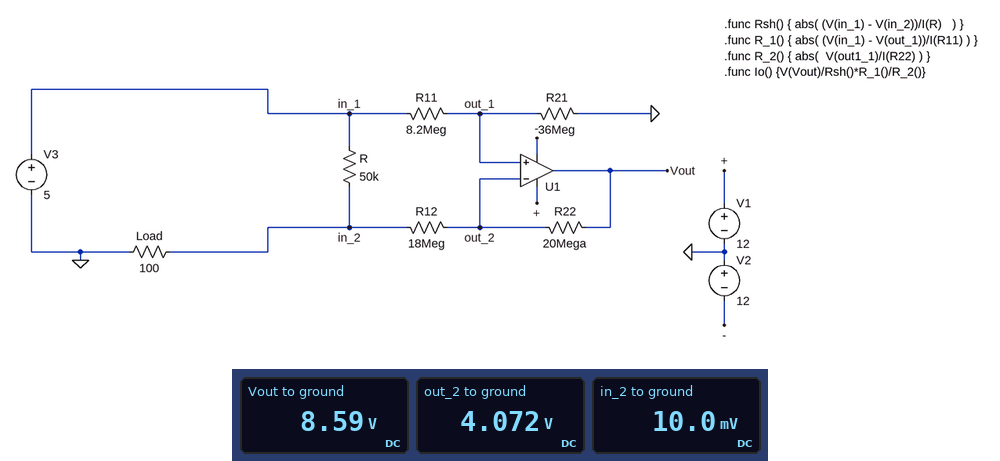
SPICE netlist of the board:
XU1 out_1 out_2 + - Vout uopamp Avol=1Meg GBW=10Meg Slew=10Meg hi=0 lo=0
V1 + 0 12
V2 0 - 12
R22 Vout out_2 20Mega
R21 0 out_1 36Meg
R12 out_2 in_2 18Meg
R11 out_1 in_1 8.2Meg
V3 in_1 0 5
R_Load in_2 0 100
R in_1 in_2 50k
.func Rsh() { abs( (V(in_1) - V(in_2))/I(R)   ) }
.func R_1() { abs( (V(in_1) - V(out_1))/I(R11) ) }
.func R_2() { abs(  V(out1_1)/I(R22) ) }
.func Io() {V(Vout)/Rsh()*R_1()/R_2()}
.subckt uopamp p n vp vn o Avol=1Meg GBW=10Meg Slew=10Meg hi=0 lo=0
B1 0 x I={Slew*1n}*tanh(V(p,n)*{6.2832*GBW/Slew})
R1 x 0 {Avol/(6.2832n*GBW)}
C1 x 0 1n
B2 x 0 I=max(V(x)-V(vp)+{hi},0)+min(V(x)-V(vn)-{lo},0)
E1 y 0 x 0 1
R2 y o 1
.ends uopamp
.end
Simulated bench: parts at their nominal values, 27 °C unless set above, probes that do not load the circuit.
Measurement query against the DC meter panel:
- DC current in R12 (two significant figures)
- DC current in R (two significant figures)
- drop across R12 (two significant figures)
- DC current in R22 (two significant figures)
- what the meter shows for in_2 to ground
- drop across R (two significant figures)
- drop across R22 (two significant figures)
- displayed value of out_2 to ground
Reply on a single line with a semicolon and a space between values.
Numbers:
230 nA; 100 µA; 4.1 V; 230 nA; 10.0 mV; 5.0 V; 4.5 V; 4.072 V
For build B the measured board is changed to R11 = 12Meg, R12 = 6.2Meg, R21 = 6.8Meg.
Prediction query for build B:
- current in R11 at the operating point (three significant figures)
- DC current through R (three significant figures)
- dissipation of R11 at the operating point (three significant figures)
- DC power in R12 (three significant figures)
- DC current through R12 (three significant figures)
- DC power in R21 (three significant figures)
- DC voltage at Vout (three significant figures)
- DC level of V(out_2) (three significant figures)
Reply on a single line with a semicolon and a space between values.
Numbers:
266 nA; 99.8 µA; 849 nW; 522 nW; 290 nA; 481 nW; 7.61 V; 1.81 V
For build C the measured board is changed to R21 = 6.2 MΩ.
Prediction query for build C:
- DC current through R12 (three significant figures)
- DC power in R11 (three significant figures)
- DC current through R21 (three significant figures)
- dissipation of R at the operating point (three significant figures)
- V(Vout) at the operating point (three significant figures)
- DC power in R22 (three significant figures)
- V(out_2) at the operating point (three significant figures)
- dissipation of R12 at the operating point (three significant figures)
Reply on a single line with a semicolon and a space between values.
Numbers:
119 nA; 989 nW; 347 nA; 498 µW; 4.53 V; 283 nW; 2.15 V; 255 nW
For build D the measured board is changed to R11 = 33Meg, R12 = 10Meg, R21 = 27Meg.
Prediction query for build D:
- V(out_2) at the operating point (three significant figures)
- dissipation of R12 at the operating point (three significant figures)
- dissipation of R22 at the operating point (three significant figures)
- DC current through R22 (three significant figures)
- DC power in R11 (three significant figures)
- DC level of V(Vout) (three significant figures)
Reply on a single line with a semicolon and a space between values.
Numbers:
2.25 V; 502 nW; 1.00 µW; 224 nA; 229 nW; 6.73 V
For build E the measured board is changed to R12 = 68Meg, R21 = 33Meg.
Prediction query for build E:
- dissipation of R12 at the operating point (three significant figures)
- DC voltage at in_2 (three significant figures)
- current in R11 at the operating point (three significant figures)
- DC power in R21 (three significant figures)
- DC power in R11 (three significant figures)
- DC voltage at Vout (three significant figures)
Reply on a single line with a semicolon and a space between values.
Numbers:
235 nW; 9.99 mV; 121 nA; 486 nW; 121 nW; 5.18 V
